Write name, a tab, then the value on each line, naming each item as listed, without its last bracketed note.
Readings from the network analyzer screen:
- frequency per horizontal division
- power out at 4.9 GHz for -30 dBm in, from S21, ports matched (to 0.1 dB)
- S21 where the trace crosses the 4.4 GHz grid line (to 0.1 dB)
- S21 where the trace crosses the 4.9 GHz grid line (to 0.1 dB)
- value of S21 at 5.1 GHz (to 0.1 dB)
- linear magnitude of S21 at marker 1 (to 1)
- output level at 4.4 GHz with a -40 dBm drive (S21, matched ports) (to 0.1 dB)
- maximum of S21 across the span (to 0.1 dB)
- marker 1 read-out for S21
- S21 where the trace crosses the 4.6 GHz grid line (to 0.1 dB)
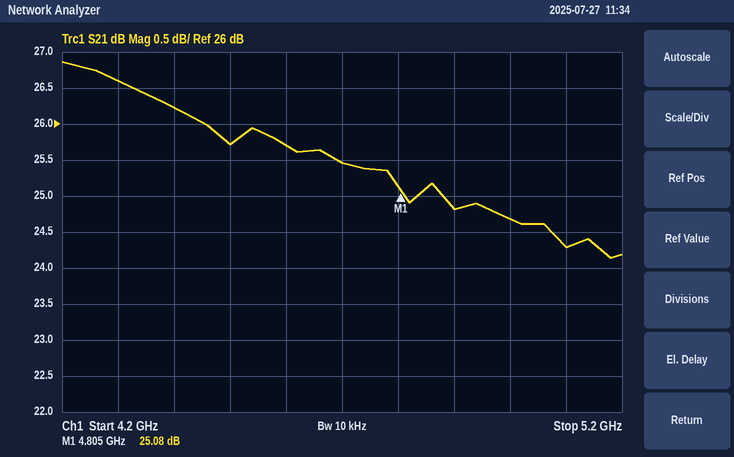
frequency per horizontal division	100 MHz
power out at 4.9 GHz for -30 dBm in, from S21, ports matched	-5.2 dBm
S21 where the trace crosses the 4.4 GHz grid line	26.2 dB
S21 where the trace crosses the 4.9 GHz grid line	24.8 dB
value of S21 at 5.1 GHz	24.3 dB
linear magnitude of S21 at marker 1	18
output level at 4.4 GHz with a -40 dBm drive (S21, matched ports)	-13.8 dBm
maximum of S21 across the span	26.9 dB
marker 1 read-out for S21	25.08 dB
S21 where the trace crosses the 4.6 GHz grid line	25.7 dB
